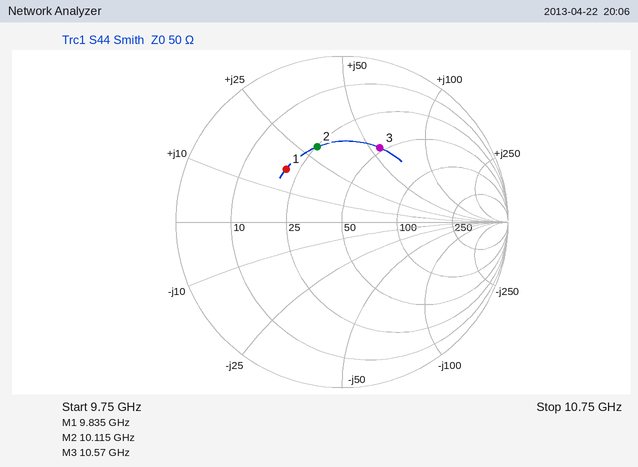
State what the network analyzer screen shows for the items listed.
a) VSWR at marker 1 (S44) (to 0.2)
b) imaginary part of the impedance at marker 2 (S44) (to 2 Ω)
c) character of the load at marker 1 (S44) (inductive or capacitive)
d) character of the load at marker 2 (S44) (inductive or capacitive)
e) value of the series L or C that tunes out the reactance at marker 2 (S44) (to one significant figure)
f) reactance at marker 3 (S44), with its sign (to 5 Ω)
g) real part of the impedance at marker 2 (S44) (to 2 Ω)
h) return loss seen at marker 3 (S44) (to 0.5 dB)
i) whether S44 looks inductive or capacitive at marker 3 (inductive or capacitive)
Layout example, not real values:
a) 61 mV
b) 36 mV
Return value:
a) 2.8
b) +30 Ω
c) inductive
d) inductive
e) 500 fF
f) +55 Ω
g) 26 Ω
h) 6.0 dB
i) inductive
